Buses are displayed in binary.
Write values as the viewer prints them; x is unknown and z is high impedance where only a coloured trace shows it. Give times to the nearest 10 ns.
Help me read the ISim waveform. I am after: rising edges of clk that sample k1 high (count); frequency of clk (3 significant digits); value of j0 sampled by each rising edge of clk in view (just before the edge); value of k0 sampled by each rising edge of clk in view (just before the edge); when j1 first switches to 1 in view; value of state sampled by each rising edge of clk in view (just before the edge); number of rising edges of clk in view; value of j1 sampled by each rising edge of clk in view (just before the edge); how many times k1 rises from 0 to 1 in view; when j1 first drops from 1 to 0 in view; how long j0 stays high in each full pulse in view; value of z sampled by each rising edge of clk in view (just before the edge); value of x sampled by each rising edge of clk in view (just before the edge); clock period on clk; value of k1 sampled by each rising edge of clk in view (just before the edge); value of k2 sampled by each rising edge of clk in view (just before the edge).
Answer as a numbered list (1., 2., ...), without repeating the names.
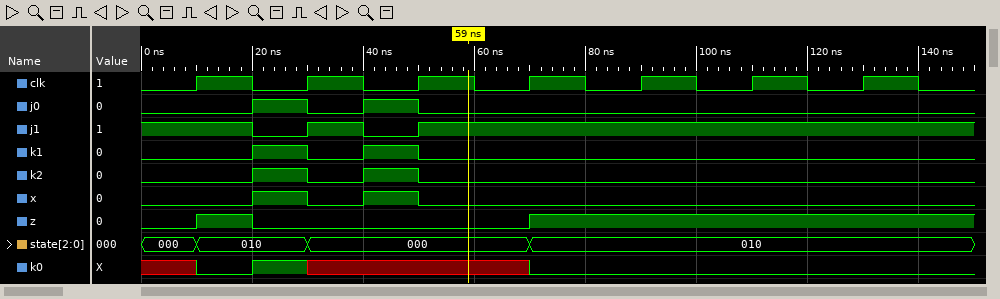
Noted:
1. 2
2. 50.0 MHz
3. 0 1 1 0 0 0 0
4. x 1 x x 0 0 0
5. 30 ns
6. 000, 010, 000, 000, 010, 010, 010
7. 7
8. 1 0 0 1 1 1 1
9. 2
10. 20 ns
11. 10 ns, 10 ns
12. 0 0 0 0 1 1 1
13. 0 1 1 0 0 0 0
14. 20 ns
15. 0 1 1 0 0 0 0
16. 0 1 1 0 0 0 0
